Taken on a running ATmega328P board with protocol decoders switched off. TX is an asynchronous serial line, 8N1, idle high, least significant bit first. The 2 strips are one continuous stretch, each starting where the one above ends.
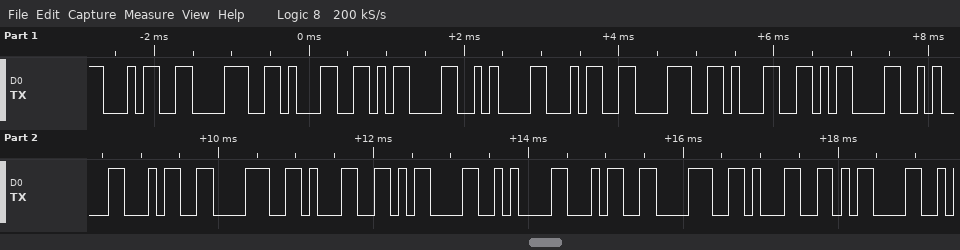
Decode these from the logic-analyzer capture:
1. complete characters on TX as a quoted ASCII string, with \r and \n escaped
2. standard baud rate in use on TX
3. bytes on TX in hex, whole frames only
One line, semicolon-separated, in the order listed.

"481\r\n481\r\n481\r\n481\r"; 9600 baud; 0x34 0x38 0x31 0x0D 0x0A 0x34 0x38 0x31 0x0D 0x0A 0x34 0x38 0x31 0x0D 0x0A 0x34 0x38 0x31 0x0D
